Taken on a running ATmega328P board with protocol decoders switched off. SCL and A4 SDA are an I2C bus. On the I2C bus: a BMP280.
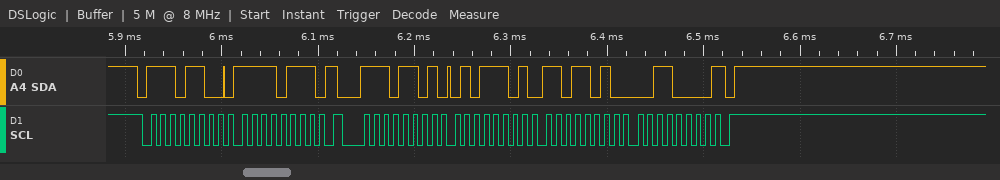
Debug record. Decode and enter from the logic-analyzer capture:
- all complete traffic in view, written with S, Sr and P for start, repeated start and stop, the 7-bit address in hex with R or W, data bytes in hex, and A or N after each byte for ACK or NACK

S 76W A F7 A Sr 76R A 5D A DA A 30 N P
